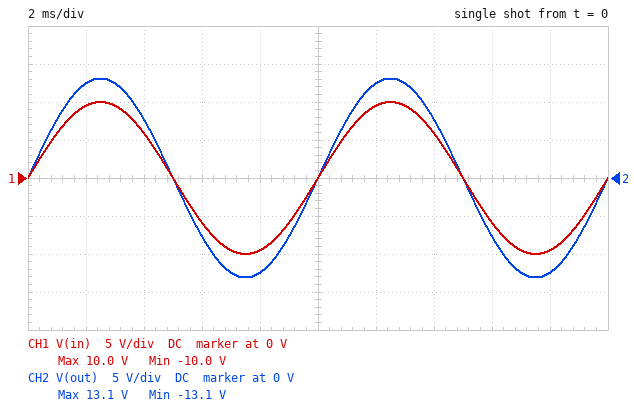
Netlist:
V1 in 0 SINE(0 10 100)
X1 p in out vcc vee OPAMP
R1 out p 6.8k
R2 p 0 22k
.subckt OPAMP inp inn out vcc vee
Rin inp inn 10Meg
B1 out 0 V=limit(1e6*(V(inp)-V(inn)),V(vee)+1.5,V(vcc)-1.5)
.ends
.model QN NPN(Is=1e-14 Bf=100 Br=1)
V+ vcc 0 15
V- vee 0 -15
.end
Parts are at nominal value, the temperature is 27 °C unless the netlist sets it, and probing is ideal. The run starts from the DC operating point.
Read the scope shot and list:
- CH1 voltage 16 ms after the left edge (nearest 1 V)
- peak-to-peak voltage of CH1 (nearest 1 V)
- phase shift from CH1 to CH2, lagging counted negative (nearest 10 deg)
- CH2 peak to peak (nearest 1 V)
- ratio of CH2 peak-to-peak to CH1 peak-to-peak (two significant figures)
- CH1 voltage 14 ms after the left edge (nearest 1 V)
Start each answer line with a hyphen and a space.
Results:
- -6 V
- 20 V
- 0 deg
- 26 V
- 1.3
- 6 V
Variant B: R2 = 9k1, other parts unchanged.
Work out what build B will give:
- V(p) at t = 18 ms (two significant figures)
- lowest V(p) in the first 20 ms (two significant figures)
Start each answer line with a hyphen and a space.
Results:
- 7.7 V
- -7.7 V
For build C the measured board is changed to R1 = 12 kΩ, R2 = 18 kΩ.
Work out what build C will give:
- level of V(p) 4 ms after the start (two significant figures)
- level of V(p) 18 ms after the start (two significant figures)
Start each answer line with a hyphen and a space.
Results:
- -8.1 V
- 8.1 V
